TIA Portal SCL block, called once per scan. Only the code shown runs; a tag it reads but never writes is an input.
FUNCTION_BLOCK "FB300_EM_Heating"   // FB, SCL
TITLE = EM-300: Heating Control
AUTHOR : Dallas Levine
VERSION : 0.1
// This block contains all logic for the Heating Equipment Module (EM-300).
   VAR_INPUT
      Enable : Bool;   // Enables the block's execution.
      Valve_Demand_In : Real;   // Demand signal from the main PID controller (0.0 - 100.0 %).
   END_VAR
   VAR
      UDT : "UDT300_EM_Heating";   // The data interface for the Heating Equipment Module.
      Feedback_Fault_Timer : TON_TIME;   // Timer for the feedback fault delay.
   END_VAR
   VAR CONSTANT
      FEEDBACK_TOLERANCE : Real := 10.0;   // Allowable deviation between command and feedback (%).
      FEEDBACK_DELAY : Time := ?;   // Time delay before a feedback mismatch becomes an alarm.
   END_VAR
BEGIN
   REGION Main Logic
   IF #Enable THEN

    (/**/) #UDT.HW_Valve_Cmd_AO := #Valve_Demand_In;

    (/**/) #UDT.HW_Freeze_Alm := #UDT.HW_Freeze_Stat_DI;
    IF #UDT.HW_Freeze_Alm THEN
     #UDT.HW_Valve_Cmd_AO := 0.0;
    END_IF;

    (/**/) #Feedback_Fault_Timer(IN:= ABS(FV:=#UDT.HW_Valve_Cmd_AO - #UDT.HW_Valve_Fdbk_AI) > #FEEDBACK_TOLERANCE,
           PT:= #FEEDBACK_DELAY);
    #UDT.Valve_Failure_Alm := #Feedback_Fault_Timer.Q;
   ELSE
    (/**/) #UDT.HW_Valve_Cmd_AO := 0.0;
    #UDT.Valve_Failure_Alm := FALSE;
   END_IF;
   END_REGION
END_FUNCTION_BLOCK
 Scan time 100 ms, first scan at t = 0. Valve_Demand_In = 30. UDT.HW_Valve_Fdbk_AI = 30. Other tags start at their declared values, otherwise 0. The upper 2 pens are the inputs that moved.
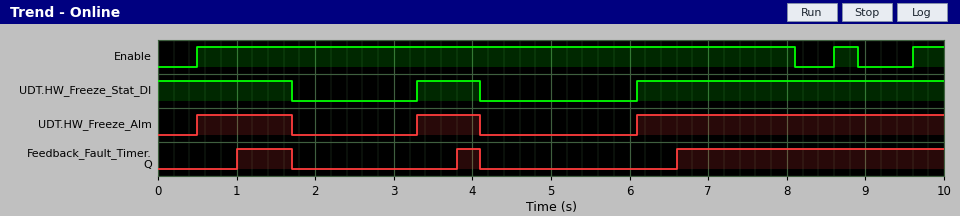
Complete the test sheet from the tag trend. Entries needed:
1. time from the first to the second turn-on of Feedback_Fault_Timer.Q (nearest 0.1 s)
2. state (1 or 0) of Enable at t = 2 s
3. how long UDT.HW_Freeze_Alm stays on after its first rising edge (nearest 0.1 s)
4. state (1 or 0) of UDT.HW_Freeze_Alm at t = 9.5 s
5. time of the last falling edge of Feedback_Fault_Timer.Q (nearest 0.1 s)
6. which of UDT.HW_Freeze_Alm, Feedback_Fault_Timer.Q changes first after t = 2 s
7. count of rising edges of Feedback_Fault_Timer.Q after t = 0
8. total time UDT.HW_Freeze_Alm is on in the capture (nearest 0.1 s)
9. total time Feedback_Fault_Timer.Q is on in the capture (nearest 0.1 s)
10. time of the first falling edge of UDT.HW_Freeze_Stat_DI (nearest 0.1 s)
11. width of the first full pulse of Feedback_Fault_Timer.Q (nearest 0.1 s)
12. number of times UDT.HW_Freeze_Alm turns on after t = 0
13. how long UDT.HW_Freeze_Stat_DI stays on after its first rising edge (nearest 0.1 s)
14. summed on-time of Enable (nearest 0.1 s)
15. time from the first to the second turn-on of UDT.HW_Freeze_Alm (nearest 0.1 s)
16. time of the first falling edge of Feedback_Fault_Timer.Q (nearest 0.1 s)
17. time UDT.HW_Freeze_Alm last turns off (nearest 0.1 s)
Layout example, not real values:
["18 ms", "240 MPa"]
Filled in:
["2.8 s", "1", "1.2 s", "1", "4.1 s", "UDT.HW_Freeze_Alm", "3", "5.9 s", "4.4 s", "1.7 s", "0.7 s", "3", "0.8 s", "8.3 s", "2.8 s", "1.7 s", "4.1 s"]
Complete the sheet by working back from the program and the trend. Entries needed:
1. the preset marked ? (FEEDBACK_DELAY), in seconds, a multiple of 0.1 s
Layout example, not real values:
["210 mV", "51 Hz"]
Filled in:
["0.5 s"]
